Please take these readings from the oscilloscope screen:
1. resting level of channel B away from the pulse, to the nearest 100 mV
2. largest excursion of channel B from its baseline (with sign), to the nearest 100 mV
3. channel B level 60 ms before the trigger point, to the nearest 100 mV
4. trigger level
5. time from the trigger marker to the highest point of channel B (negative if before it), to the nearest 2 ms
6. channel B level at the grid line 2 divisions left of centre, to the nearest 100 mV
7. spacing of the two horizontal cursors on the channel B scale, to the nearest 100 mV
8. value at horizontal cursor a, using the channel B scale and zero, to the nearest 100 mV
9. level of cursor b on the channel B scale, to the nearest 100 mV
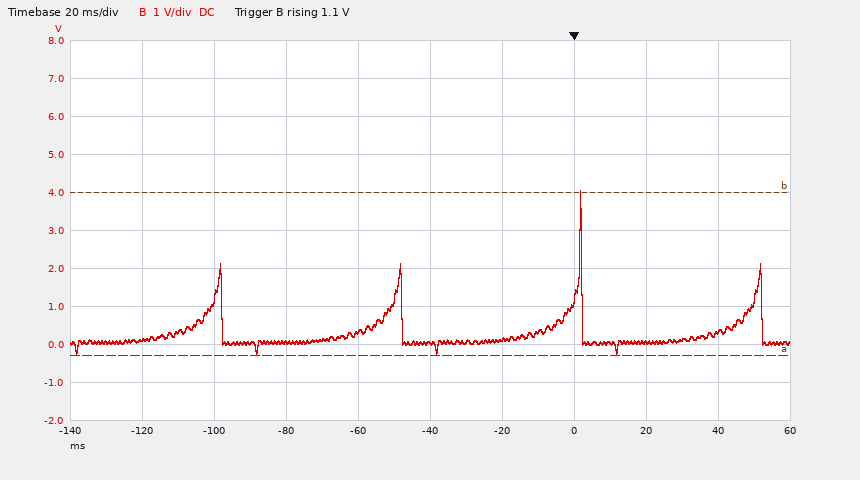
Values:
100 mV
+4.0 V
300 mV
1.1 V
+2 ms
100 mV
4.3 V
-300 mV
4.0 V
